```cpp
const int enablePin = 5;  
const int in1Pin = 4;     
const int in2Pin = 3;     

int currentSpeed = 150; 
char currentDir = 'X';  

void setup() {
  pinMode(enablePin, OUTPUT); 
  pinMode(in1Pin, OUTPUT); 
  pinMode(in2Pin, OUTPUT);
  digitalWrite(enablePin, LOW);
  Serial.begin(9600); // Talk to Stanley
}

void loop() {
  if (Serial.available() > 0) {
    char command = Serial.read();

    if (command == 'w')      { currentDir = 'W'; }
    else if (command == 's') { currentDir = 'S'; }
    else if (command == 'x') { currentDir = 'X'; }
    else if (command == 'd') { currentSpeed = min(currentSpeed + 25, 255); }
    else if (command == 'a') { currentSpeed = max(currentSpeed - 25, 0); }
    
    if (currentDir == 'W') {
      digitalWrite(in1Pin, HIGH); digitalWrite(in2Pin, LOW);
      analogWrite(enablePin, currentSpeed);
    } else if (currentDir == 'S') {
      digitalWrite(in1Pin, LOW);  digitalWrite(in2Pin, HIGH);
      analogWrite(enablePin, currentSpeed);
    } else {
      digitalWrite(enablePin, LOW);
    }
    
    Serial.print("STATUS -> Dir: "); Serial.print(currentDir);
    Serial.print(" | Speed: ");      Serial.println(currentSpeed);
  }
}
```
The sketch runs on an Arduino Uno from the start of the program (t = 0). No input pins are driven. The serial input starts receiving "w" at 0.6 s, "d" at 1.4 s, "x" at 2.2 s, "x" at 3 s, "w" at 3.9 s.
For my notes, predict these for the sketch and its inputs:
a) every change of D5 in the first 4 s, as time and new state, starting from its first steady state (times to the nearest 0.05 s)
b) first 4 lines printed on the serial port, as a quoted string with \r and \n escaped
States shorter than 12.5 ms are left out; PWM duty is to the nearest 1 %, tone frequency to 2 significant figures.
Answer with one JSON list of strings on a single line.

["0 s low; 0.6 s PWM 59 %; 1.4 s PWM 69 %; 2.2 s low; 3.9 s PWM 69 %", "\"STATUS -> Dir: W | Speed: 150\\r\\nSTATUS -> Dir: W | Speed: 175\\r\\nSTATUS -> Dir: X | Speed: 175\\r\\nSTATUS -> Dir: X | Speed: 175\\r\\n\""]
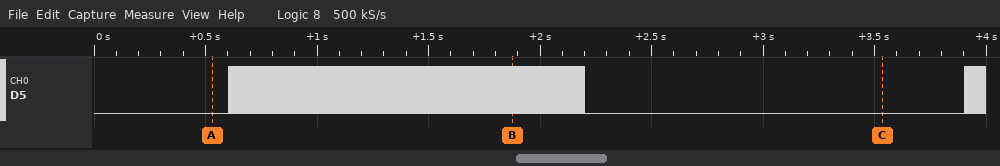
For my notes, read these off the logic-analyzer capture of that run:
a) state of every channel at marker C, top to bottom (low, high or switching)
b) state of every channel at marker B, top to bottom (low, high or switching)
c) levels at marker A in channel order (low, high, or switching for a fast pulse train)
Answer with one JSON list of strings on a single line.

["D5 low", "D5 switching", "D5 low"]
